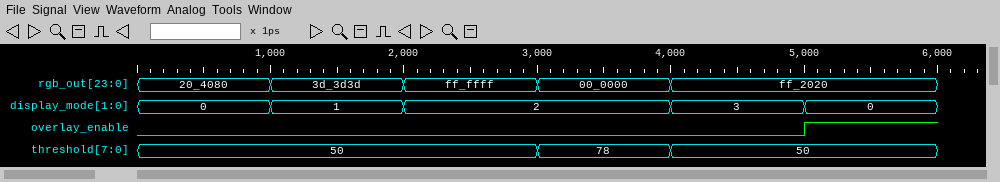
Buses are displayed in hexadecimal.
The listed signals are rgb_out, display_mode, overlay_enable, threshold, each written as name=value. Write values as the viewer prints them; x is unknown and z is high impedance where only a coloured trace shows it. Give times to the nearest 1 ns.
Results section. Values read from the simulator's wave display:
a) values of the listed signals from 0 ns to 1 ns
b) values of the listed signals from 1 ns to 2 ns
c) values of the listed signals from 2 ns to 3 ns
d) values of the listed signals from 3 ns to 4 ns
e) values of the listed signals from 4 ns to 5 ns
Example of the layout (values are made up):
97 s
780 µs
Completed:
rgb_out=20_4080, display_mode=0, overlay_enable=0, threshold=50
rgb_out=3d_3d3d, display_mode=1, overlay_enable=0, threshold=50
rgb_out=ff_ffff, display_mode=2, overlay_enable=0, threshold=50
rgb_out=00_0000, display_mode=2, overlay_enable=0, threshold=78
rgb_out=ff_2020, display_mode=3, overlay_enable=0, threshold=50
